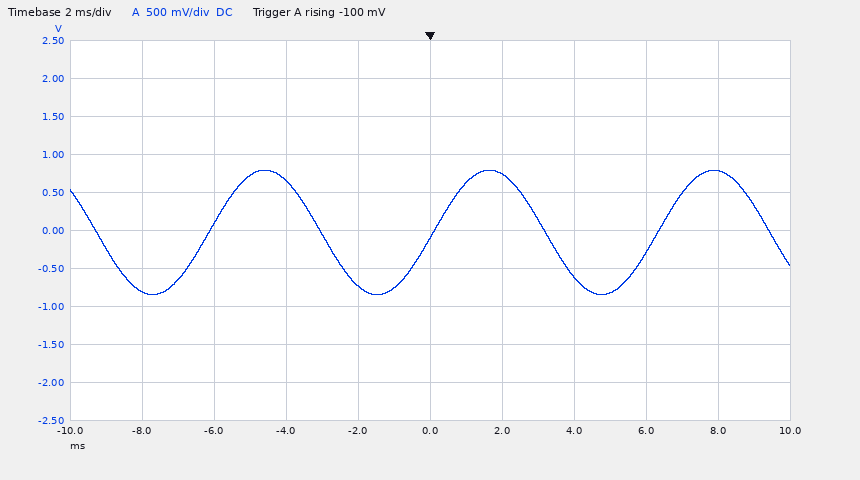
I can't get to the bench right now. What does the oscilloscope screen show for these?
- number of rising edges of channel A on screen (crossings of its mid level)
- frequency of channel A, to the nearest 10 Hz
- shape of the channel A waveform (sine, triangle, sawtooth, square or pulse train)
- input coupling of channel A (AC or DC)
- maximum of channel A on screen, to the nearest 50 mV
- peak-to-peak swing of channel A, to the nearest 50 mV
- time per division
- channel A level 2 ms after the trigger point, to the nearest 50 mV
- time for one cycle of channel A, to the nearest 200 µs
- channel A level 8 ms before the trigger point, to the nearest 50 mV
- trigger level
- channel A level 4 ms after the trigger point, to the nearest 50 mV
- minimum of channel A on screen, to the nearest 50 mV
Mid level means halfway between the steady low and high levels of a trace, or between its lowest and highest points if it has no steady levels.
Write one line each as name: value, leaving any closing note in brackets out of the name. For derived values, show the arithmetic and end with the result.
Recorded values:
number of rising edges of channel A on screen: 3
frequency of channel A, to the nearest 10 Hz: 1 / 6.2 ms ≈ 161 Hz, so 160 Hz to the nearest 10 Hz
shape of the channel A waveform: sine
input coupling of channel A: DC
maximum of channel A on screen, to the nearest 50 mV: 800 mV
peak-to-peak swing of channel A, to the nearest 50 mV: 800 mV − (-850 mV) = 1.65 V
time per division: 2 ms
channel A level 2 ms after the trigger point, to the nearest 50 mV: 750 mV
time for one cycle of channel A, to the nearest 200 µs: 6.2 ms
channel A level 8 ms before the trigger point, to the nearest 50 mV: -800 mV
trigger level: -100 mV
channel A level 4 ms after the trigger point, to the nearest 50 mV: -600 mV
minimum of channel A on screen, to the nearest 50 mV: -850 mV
